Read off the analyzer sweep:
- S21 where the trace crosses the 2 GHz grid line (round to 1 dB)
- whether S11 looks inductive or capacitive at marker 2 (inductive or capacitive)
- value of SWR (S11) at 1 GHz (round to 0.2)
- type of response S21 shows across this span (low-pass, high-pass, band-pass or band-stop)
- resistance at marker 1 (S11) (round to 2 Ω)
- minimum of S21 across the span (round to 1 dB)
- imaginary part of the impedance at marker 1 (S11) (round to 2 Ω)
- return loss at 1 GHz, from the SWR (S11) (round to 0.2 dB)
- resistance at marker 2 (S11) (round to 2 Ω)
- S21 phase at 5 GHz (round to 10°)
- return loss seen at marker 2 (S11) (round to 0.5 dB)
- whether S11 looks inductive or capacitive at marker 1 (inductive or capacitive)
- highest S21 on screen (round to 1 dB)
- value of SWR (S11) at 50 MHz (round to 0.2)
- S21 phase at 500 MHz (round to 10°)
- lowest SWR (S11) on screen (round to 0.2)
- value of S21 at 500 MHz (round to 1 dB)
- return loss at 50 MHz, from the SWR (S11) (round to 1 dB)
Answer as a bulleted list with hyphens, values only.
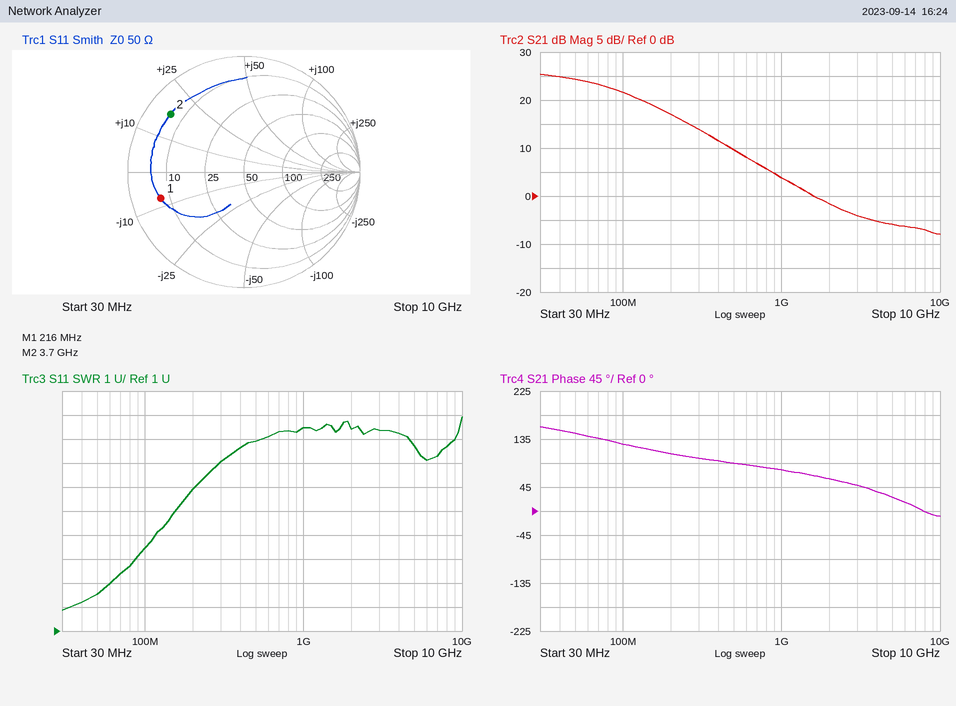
- -2 dB
- inductive
- 9.4
- low-pass
- 8 Ω
- -8 dB
- -8 Ω
- 1.8 dB
- 6 Ω
- 30°
- 2.0 dB
- capacitive
- 25 dB
- 2.6
- 90°
- 1.8
- 10 dB
- 7 dB
